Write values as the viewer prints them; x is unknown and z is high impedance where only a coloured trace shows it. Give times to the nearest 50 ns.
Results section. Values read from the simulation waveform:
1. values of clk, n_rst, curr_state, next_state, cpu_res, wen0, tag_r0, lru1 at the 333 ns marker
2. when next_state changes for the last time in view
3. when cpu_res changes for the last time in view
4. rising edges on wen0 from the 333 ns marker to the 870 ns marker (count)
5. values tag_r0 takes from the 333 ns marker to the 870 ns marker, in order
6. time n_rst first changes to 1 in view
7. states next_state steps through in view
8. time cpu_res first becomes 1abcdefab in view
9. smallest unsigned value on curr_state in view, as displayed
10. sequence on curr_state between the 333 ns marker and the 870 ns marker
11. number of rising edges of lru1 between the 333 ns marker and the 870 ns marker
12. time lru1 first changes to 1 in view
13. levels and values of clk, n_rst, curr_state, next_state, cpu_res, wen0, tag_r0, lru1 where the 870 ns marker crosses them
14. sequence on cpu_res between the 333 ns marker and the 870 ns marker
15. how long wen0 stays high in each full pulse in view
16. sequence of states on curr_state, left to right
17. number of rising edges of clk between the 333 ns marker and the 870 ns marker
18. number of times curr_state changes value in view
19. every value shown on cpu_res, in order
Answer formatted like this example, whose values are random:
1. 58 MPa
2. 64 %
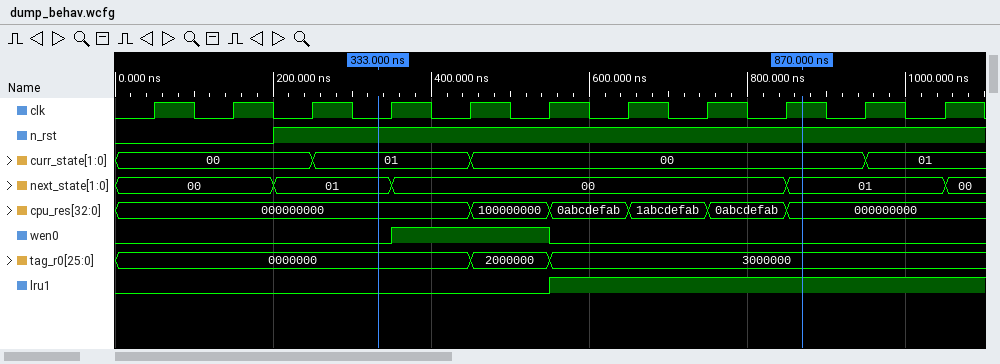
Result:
1. clk=0, n_rst=1, curr_state=01, next_state=01, cpu_res=000000000, wen0=0, tag_r0=0000000, lru1=0
2. 1050 ns
3. 850 ns
4. 1
5. 0000000, 2000000, 3000000
6. 200 ns
7. 00, 01, 00, 01, 00
8. 650 ns
9. 00
10. 01, 00
11. 1
12. 550 ns
13. clk=1, n_rst=1, curr_state=00, next_state=01, cpu_res=000000000, wen0=0, tag_r0=3000000, lru1=1
14. 000000000, 100000000, 0abcdefab, 1abcdefab, 0abcdefab, 000000000
15. 200 ns
16. 00, 01, 00, 01
17. 6
18. 3
19. 000000000, 100000000, 0abcdefab, 1abcdefab, 0abcdefab, 000000000
